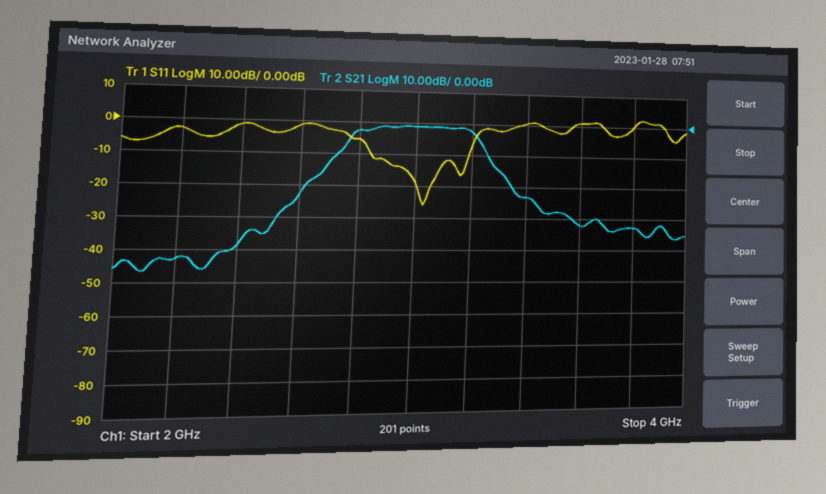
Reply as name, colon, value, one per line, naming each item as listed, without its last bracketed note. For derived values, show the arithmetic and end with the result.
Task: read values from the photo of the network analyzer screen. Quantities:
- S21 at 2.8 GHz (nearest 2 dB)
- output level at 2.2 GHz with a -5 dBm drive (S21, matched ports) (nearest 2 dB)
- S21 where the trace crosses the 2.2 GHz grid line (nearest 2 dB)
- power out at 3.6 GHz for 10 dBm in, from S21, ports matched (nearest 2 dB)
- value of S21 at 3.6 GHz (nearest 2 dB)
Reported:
S21 at 2.8 GHz: -2 dB
output level at 2.2 GHz with a -5 dBm drive (S21, matched ports): -5 dBm + (-42 dB) = -48 dBm
S21 where the trace crosses the 2.2 GHz grid line: -42 dB
power out at 3.6 GHz for 10 dBm in, from S21, ports matched: 10 dBm + (-32 dB) = -22 dBm
value of S21 at 3.6 GHz: -32 dB
